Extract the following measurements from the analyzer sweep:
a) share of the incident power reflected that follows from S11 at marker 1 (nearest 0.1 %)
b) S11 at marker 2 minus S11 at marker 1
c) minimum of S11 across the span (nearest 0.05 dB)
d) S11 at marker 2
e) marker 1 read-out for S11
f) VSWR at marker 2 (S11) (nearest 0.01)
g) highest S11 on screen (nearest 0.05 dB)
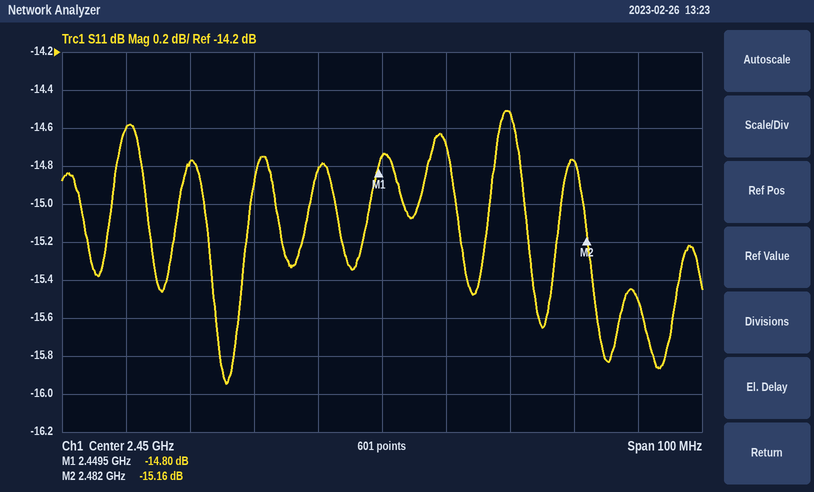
3.3 %
-0.36 dB
-15.95 dB
-15.16 dB
-14.80 dB
1.42
-14.50 dB
